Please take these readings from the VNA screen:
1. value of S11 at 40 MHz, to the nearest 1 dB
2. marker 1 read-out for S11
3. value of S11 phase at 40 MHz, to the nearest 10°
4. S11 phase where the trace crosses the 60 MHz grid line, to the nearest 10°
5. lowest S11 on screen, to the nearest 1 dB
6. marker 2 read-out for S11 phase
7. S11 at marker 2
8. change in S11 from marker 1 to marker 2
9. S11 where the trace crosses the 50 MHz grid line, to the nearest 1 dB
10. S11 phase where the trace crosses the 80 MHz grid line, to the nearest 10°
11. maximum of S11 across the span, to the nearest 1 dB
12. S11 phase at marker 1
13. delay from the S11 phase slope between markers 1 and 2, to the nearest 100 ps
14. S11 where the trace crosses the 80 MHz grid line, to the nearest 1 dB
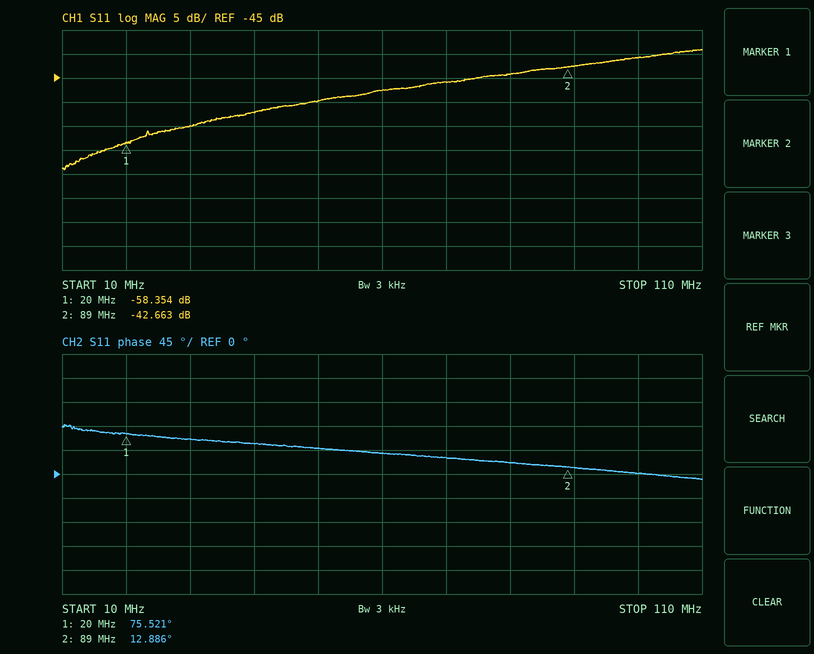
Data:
-52 dB
-58.354 dB
60°
40°
-64 dB
12.886°
-42.663 dB
15.691 dB
-50 dB
20°
-39 dB
75.521°
2.5 ns
-44 dB
